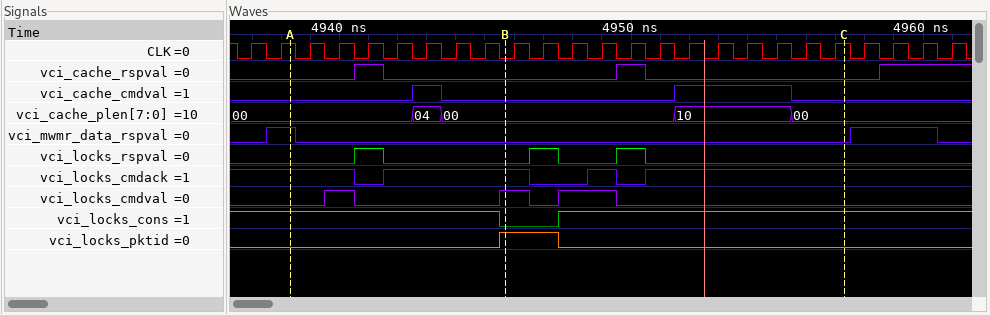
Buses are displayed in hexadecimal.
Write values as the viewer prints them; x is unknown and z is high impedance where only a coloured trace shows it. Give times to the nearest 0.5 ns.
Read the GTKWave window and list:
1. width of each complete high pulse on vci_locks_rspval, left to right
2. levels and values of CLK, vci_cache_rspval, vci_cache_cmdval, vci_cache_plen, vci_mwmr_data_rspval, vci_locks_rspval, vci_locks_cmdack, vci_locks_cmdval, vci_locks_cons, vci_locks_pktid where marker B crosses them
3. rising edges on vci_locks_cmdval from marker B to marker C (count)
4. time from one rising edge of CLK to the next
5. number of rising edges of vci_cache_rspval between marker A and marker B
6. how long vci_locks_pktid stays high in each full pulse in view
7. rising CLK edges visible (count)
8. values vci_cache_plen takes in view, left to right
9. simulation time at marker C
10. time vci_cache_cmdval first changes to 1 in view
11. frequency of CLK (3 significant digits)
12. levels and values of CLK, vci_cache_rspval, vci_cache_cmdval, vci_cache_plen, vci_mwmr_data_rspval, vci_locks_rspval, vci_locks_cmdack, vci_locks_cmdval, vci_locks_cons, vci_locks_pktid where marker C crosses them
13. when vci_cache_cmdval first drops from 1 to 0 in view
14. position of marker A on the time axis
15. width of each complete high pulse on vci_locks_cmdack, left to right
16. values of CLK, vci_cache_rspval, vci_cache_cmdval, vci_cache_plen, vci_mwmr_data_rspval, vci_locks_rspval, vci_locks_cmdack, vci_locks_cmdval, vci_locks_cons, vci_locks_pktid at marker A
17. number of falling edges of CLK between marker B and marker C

1 ns, 1 ns, 1 ns
CLK=0, vci_cache_rspval=0, vci_cache_cmdval=0, vci_cache_plen=00, vci_mwmr_data_rspval=0, vci_locks_rspval=0, vci_locks_cmdack=1, vci_locks_cmdval=1, vci_locks_cons=0, vci_locks_pktid=1
1
1 ns
1
2 ns
25
00, 04, 00, 10, 00
4957.5 ns
4942.5 ns
1.00 GHz
CLK=1, vci_cache_rspval=0, vci_cache_cmdval=0, vci_cache_plen=00, vci_mwmr_data_rspval=0, vci_locks_rspval=0, vci_locks_cmdack=1, vci_locks_cmdval=0, vci_locks_cons=1, vci_locks_pktid=0
4943.5 ns
4938.5 ns
5 ns, 1 ns
CLK=1, vci_cache_rspval=0, vci_cache_cmdval=0, vci_cache_plen=00, vci_mwmr_data_rspval=1, vci_locks_rspval=0, vci_locks_cmdack=1, vci_locks_cmdval=0, vci_locks_cons=1, vci_locks_pktid=0
11
